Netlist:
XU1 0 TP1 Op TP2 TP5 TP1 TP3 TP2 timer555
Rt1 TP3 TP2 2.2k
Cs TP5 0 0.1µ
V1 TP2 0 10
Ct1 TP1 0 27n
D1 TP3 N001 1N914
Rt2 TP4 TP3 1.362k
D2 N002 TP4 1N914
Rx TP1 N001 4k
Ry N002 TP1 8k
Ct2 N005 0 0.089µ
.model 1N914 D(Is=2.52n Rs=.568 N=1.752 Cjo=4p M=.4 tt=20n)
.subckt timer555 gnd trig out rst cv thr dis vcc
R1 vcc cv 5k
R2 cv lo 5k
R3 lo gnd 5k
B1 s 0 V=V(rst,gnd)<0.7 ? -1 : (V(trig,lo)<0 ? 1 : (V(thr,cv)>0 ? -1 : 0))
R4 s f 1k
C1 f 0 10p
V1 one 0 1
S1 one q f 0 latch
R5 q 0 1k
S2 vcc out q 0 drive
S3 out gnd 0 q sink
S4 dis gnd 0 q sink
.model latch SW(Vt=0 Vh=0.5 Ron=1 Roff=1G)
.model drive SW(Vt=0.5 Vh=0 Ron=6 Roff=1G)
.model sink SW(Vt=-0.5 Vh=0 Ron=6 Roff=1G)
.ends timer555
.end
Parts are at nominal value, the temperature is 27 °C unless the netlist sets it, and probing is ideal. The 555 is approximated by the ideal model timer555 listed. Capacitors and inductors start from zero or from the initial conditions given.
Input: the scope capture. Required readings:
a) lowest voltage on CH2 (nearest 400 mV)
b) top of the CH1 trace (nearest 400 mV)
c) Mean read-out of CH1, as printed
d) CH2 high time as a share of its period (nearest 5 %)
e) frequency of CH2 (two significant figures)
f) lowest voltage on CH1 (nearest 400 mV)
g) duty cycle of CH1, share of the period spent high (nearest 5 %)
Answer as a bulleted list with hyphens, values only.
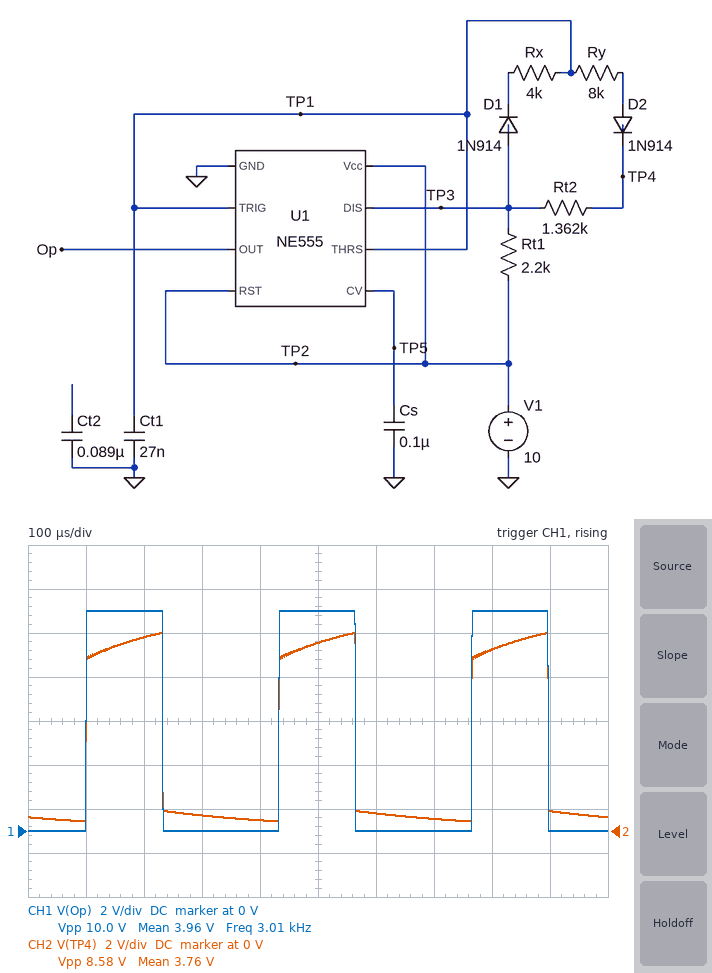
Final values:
- 400 mV
- 10.0 V
- 3.96 V
- 40 %
- 3.0 kHz
- 0 V
- 40 %
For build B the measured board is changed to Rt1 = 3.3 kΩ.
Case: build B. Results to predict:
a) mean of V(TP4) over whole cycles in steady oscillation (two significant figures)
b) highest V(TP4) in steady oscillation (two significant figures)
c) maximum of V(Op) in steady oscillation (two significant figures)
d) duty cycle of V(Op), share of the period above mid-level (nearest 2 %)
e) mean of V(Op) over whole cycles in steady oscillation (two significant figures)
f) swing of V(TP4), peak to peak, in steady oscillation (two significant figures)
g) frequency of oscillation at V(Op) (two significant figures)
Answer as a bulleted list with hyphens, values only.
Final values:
- 3.9 V
- 8.7 V
- 10 V
- 44 %
- 4.4 V
- 8.3 V
- 2.8 kHz
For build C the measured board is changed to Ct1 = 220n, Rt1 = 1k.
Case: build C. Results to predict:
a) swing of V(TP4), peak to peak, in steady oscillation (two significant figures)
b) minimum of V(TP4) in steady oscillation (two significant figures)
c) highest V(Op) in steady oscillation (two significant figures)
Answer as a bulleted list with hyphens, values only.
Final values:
- 9.0 V
- 460 mV
- 10 V
